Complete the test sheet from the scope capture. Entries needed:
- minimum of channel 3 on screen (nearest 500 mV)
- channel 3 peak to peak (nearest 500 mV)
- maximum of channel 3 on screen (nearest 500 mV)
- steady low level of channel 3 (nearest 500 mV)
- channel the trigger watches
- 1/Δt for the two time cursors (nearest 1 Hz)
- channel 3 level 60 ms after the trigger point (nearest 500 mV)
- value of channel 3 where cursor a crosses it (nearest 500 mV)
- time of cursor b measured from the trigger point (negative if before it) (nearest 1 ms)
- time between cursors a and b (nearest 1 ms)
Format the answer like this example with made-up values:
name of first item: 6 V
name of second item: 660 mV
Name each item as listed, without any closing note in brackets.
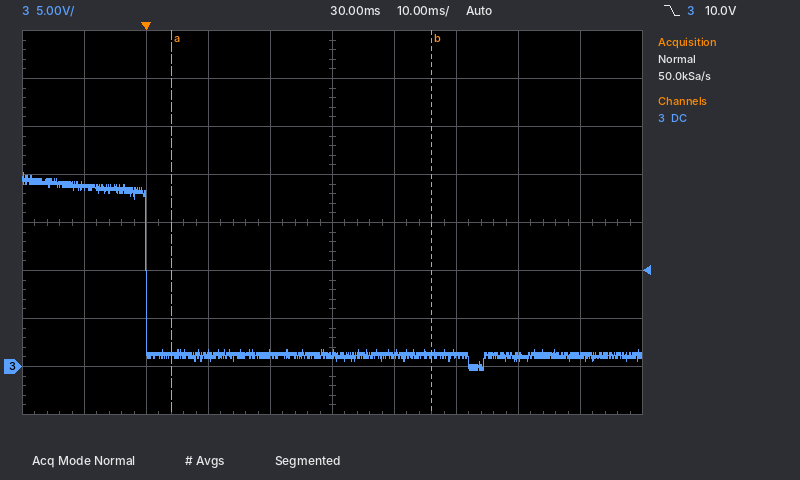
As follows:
minimum of channel 3 on screen: -500 mV
channel 3 peak to peak: 20.5 V
maximum of channel 3 on screen: 20.0 V
steady low level of channel 3: 1.0 V
channel the trigger watches: channel 3
1/Δt for the two time cursors: 24 Hz
channel 3 level 60 ms after the trigger point: 1.0 V
value of channel 3 where cursor a crosses it: 1.0 V
time of cursor b measured from the trigger point (negative if before it): +46 ms
time between cursors a and b: 42 ms
